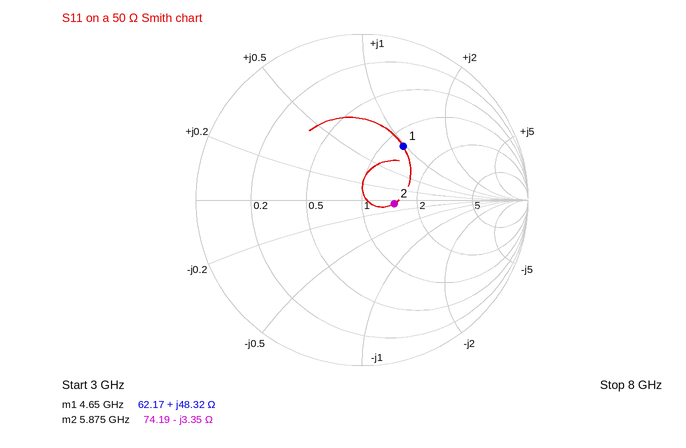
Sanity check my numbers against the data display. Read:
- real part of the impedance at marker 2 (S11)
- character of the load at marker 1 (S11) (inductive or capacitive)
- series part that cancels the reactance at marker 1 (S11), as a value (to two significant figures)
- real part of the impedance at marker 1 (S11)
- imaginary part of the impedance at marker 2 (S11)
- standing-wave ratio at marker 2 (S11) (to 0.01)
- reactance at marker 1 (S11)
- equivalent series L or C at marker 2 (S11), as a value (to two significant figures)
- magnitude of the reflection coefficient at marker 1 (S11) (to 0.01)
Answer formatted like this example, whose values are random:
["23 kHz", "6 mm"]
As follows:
["74.19 Ω", "inductive", "710 fF", "62.17 Ω", "-3.35 Ω", "1.49", "+48.32 Ω", "8.1 pF", "0.41"]
